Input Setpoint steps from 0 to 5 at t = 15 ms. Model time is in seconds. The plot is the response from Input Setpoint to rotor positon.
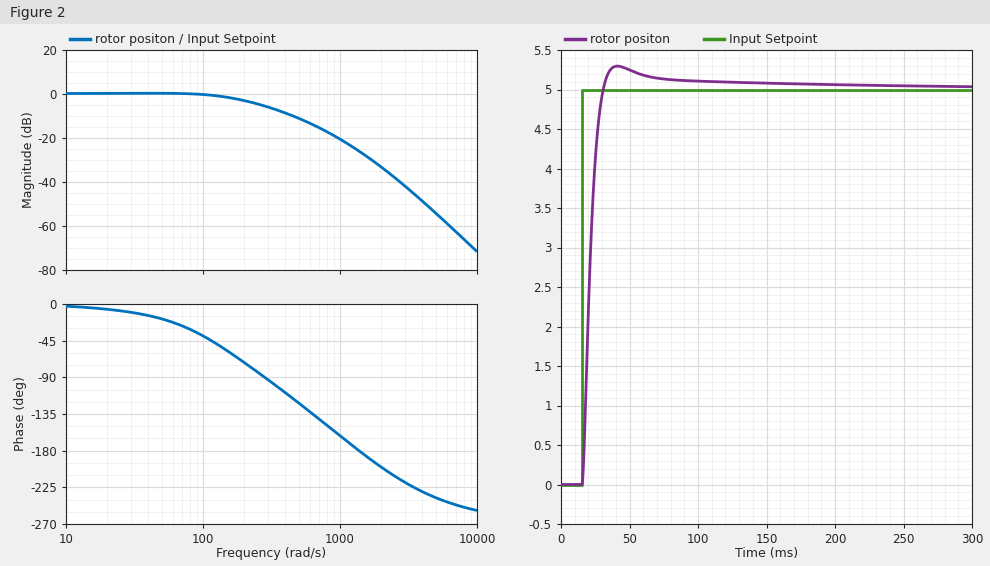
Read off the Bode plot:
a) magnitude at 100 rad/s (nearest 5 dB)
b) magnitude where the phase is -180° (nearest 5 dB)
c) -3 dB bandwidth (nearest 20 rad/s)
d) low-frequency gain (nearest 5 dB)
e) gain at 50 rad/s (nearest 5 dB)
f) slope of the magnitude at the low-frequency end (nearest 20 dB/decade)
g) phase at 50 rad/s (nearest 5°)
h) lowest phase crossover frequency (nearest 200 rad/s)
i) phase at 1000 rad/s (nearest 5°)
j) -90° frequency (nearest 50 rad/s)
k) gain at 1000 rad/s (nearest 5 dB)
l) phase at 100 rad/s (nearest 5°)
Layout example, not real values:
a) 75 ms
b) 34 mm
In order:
a) 0 dB
b) -25 dB
c) 200 rad/s
d) 0 dB
e) 0 dB
f) 0 dB/decade
g) -20°
h) 1400 rad/s
i) -160°
j) 300 rad/s
k) -20 dB
l) -40°
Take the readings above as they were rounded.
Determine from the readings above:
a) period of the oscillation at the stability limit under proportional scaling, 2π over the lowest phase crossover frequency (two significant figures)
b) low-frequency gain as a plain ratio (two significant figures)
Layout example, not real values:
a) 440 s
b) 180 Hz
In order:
a) 0.0045 s
b) 1.0
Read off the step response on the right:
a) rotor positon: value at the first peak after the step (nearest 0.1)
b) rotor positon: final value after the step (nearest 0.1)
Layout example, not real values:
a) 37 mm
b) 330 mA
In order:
a) 5.3
b) 5.0
